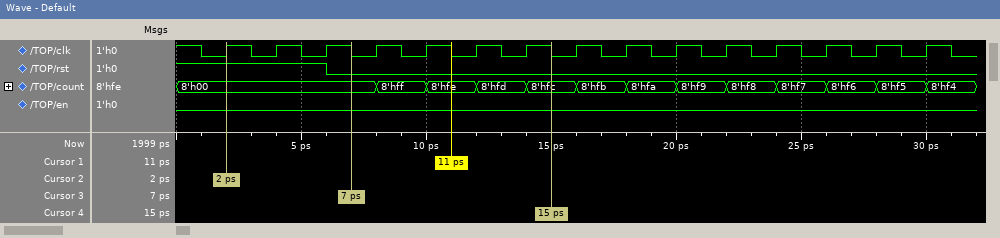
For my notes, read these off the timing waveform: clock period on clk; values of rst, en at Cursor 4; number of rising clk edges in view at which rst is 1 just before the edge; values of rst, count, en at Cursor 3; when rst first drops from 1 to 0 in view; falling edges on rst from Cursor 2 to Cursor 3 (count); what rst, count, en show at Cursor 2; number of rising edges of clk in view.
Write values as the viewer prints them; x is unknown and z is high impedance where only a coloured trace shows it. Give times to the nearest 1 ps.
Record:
2 ps
rst=0, en=0
3
rst=0, count=8'h00, en=0
6 ps
1
rst=1, count=8'h00, en=0
15
